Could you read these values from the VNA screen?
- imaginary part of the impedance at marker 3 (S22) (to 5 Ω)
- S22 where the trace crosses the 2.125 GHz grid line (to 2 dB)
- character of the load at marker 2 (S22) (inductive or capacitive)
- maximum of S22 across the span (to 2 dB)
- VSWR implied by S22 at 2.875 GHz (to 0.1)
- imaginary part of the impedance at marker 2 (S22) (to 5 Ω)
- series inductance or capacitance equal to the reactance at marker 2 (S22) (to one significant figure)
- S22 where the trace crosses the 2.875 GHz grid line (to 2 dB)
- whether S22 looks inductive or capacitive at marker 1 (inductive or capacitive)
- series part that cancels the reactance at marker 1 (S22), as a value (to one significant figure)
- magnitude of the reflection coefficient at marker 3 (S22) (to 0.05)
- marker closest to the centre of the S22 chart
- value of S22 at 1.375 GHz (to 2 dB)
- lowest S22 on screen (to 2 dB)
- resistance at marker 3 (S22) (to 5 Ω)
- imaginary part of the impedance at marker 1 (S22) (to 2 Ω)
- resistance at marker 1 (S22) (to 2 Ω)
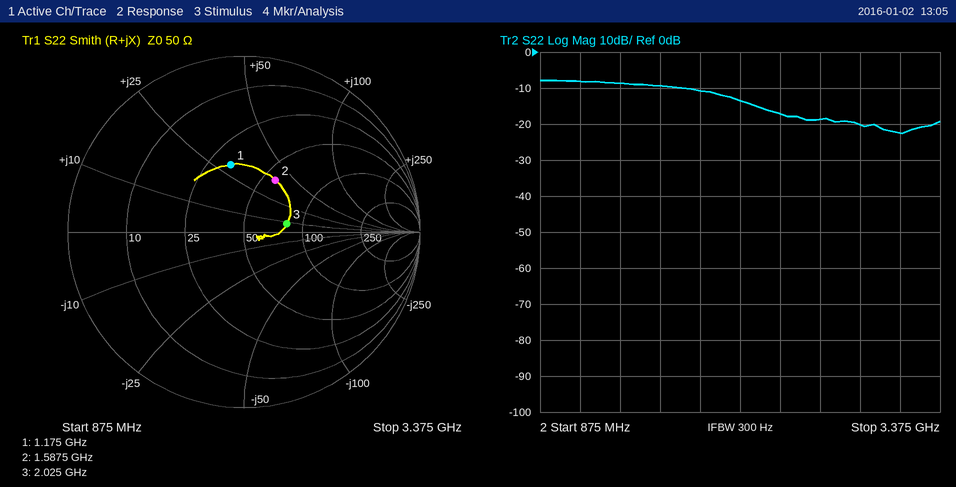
+10 Ω
-14 dB
inductive
-8 dB
1.2
+40 Ω
4 nH
-20 dB
inductive
5 pF
0.25
marker 3
-8 dB
-22 dB
80 Ω
+30 Ω
32 Ω
